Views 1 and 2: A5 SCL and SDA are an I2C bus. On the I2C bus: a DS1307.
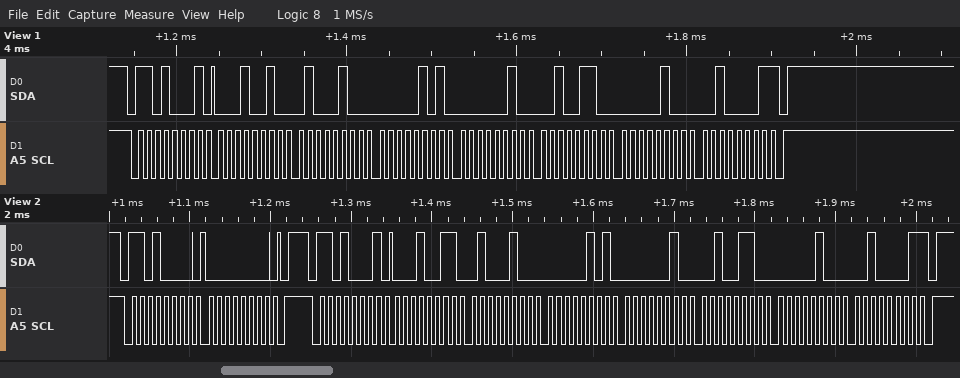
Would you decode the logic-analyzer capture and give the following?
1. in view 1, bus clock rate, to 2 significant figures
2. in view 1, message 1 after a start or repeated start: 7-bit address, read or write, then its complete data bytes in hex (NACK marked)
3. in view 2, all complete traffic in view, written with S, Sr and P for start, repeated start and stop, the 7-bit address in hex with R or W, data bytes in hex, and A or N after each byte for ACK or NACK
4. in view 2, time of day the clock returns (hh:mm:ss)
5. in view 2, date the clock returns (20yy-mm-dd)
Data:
100 kHz
0x68 read: 12 44 05 02 26 04 21 NACK
S 68W A 00 A P S 68R A 13 A 44 A 05 A 02 A 26 A 04 A 21 N P
05:44:13
2021-04-26
